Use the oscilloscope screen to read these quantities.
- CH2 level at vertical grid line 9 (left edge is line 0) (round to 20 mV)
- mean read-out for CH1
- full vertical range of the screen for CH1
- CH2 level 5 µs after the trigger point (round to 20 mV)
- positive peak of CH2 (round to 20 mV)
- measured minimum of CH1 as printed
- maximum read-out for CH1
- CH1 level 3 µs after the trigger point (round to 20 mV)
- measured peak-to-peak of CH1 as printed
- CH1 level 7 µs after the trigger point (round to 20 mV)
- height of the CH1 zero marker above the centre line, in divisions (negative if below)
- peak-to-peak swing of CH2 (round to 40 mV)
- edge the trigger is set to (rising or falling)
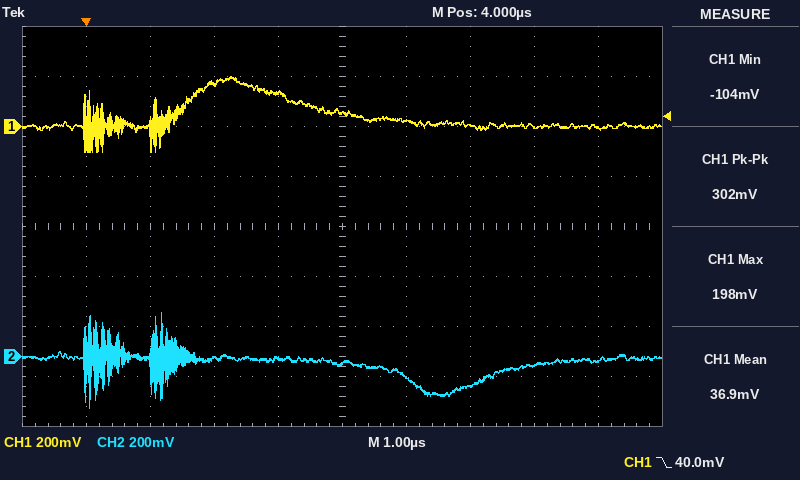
-20 mV
36.9 mV
1.6 V
-80 mV
180 mV
-104 mV
198 mV
140 mV
302 mV
0 mV
+2.0 div
400 mV
falling
